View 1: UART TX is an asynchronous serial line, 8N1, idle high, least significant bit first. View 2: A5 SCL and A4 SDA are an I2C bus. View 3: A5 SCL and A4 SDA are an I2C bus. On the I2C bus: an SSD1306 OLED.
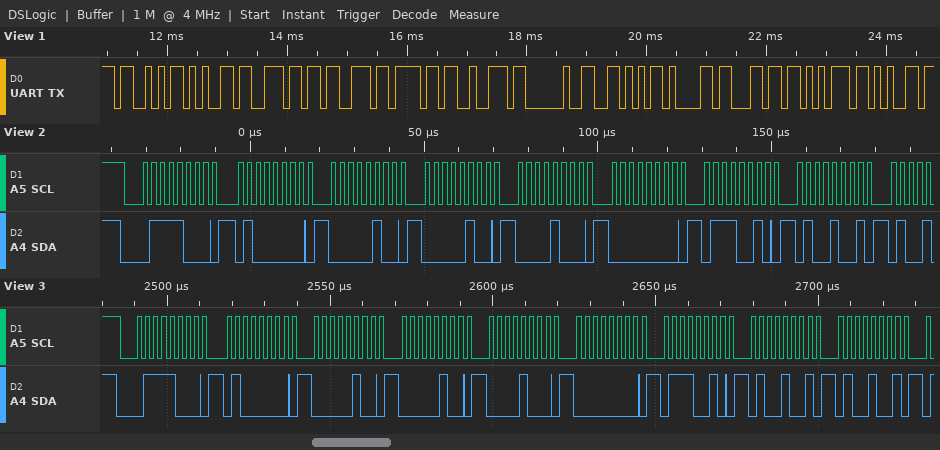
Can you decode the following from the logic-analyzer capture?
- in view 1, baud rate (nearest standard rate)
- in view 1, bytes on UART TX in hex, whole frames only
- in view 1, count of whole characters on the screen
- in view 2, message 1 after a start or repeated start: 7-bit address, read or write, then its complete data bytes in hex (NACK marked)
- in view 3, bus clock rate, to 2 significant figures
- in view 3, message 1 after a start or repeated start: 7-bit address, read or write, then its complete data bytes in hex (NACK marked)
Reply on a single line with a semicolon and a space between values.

9600 baud; 53 65 6E 73 6F 72 20 56 61 6C 75 65; 12; 0x3C write: 40 04 04 08 00 72 49; 400 kHz; 0x3C write: 40 04 04 08 00 72 49 49
